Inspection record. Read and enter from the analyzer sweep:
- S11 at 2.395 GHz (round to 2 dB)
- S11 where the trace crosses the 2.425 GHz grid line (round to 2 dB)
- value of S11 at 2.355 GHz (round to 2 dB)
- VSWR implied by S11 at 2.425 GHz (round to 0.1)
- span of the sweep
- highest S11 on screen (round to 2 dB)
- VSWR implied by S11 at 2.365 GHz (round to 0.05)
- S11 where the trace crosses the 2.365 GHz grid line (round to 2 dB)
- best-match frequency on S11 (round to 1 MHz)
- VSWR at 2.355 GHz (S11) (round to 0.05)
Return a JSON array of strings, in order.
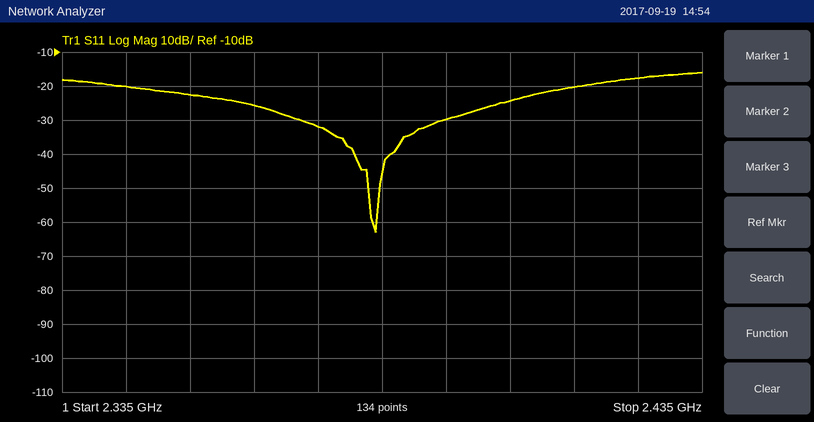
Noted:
["-30 dB", "-18 dB", "-22 dB", "1.3", "100 MHz", "-16 dB", "1.10", "-26 dB", "2.384 GHz", "1.15"]
